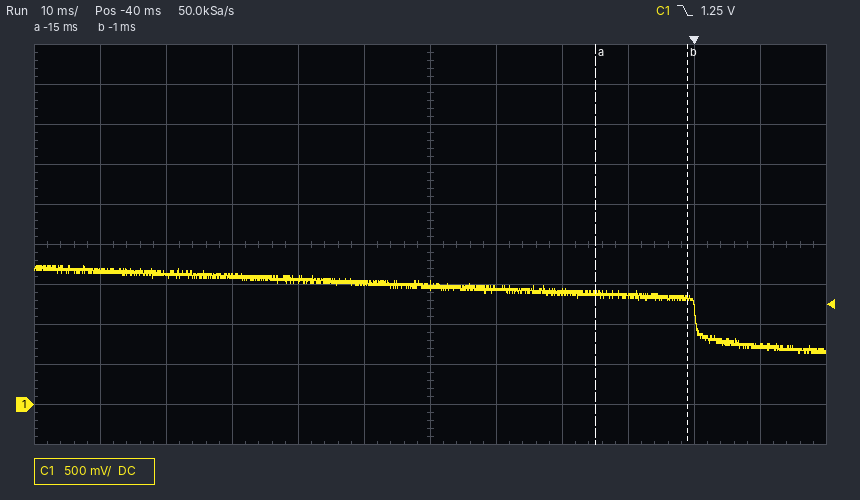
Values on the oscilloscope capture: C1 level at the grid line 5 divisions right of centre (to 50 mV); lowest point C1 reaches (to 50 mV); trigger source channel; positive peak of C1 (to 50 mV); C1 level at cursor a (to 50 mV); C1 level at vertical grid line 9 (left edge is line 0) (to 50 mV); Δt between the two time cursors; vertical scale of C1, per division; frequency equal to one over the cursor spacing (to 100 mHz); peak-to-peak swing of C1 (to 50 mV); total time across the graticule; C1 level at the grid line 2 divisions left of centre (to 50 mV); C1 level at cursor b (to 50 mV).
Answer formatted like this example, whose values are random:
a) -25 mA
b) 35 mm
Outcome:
a) 750 mV
b) 650 mV
c) C1
d) 1.75 V
e) 1.40 V
f) 1.35 V
g) 14 ms
h) 500 mV
i) 71.4 Hz
j) 1.10 V
k) 120 ms
l) 1.55 V
m) 1.35 V
